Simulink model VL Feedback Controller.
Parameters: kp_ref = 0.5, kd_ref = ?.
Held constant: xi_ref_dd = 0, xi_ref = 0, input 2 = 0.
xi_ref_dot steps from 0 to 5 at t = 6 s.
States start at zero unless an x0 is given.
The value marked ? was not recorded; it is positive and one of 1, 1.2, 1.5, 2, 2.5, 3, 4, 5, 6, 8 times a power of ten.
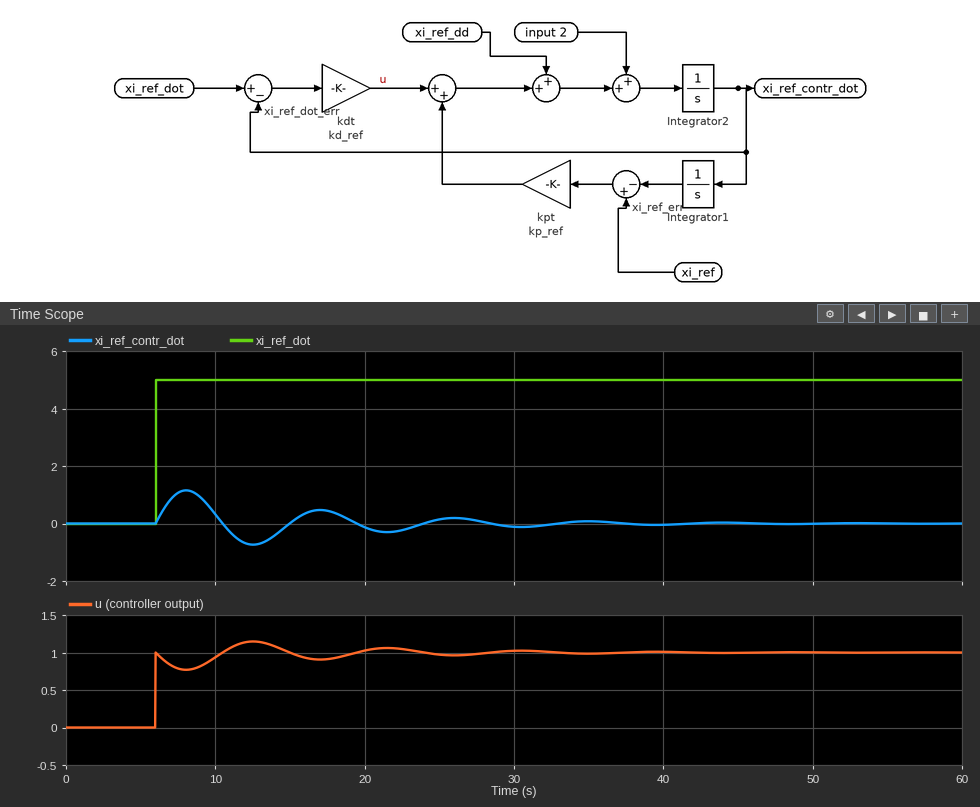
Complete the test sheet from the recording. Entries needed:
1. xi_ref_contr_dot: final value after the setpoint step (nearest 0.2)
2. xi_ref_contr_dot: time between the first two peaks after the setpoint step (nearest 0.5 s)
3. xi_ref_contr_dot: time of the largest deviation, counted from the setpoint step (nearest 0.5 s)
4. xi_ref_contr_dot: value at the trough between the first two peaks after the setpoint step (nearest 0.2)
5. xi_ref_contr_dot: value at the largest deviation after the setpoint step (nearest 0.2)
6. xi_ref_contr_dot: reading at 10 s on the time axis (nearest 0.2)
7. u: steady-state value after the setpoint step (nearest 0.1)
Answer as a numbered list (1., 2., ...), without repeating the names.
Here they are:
1. 0.0
2. 9.0 s
3. 2.0 s
4. -0.8
5. 1.2
6. 0.4
7. 1.0
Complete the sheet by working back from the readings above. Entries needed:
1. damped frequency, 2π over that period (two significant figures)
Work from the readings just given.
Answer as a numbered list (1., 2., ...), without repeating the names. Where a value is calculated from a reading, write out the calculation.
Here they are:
1. 2π / 9 = 0.70 rad/s
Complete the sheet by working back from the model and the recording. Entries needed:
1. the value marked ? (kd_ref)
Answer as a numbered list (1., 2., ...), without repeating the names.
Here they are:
1. 0.2
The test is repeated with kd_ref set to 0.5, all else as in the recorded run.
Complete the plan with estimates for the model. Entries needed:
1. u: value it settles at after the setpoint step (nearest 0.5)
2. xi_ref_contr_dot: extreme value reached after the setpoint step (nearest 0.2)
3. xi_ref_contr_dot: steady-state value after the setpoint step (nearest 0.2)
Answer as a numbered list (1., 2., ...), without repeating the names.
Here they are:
1. 2.5
2. 2.2
3. 0.0
